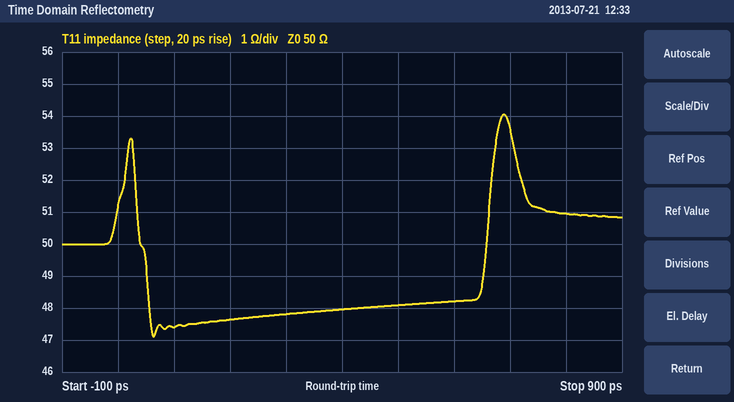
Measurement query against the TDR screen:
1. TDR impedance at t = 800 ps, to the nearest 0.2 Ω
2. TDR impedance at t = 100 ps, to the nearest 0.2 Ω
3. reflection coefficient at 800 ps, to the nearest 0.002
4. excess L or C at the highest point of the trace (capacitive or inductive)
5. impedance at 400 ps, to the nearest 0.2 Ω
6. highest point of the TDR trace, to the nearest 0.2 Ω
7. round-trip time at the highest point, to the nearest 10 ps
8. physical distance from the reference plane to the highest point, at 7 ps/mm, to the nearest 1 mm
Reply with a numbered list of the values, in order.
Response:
1. 51.0 Ω
2. 47.4 Ω
3. +0.010
4. inductive
5. 48.0 Ω
6. 54.0 Ω
7. 690 ps
8. 49 mm
